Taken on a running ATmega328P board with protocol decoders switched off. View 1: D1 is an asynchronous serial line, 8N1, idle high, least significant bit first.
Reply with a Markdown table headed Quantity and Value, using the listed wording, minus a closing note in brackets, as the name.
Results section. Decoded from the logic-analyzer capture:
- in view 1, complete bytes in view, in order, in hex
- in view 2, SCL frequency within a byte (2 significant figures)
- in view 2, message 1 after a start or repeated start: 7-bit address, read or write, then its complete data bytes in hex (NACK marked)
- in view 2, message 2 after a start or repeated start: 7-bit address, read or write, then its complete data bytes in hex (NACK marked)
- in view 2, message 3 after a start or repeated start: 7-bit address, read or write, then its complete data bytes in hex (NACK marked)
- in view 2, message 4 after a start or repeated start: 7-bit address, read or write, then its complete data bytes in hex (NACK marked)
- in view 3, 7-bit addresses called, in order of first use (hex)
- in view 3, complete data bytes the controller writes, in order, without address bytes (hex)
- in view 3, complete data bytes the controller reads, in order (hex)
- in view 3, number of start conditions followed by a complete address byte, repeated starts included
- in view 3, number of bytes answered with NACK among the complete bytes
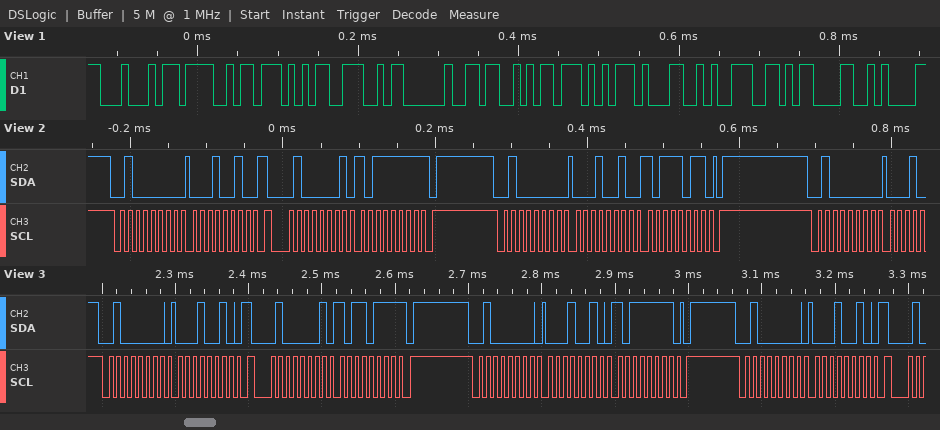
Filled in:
| Quantity | Value |
|---|---|
| in view 1, complete bytes in view, in order, in hex | 44 4F 57 4E 20 53 57 31 39 0D 0A |
| in view 2, SCL frequency within a byte | 100 kHz |
| in view 2, message 1 after a start or repeated start: 7-bit address, read or write, then its complete data bytes in hex | 0x20 write: 12 |
| in view 2, message 2 after a start or repeated start: 7-bit address, read or write, then its complete data bytes in hex | 0x20 read: BF NACK |
| in view 2, message 3 after a start or repeated start: 7-bit address, read or write, then its complete data bytes in hex | 0x20 write: 12 BB |
| in view 2, message 4 after a start or repeated start: 7-bit address, read or write, then its complete data bytes in hex | 0x20 write |
| in view 3, 7-bit addresses called, in order of first use | 0x20 |
| in view 3, complete data bytes the controller writes, in order, without address bytes | 12 12 BF 12 |
| in view 3, complete data bytes the controller reads, in order | B7 |
| in view 3, number of start conditions followed by a complete address byte, repeated starts included | 4 |
| in view 3, number of bytes answered with NACK among the complete bytes | 1 |
